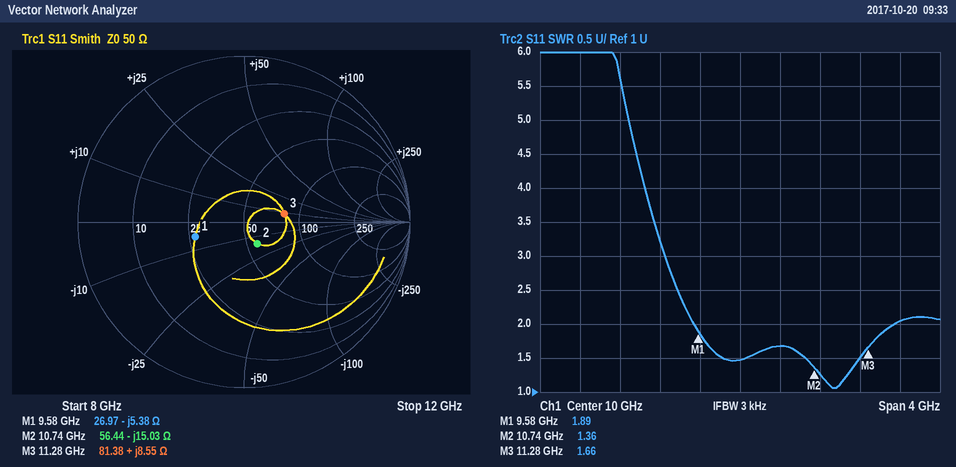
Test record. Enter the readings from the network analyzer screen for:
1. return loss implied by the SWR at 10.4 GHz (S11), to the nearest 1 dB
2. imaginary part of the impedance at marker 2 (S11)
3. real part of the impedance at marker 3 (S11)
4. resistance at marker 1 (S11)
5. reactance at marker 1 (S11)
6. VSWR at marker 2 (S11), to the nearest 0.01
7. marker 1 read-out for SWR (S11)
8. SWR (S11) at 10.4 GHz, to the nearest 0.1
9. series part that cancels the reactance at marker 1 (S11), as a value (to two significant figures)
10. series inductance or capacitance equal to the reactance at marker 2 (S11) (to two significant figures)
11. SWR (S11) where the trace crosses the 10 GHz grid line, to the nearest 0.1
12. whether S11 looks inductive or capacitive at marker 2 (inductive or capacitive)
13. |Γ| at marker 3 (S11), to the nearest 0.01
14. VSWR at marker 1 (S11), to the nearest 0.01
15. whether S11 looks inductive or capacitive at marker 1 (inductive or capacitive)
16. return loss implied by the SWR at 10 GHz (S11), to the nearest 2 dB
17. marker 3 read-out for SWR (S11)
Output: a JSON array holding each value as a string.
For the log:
["12 dB", "-15.03 Ω", "81.38 Ω", "26.97 Ω", "-5.38 Ω", "1.36", "1.89", "1.7", "89 pH", "990 fF", "1.5", "capacitive", "0.25", "1.88", "capacitive", "14 dB", "1.66"]
